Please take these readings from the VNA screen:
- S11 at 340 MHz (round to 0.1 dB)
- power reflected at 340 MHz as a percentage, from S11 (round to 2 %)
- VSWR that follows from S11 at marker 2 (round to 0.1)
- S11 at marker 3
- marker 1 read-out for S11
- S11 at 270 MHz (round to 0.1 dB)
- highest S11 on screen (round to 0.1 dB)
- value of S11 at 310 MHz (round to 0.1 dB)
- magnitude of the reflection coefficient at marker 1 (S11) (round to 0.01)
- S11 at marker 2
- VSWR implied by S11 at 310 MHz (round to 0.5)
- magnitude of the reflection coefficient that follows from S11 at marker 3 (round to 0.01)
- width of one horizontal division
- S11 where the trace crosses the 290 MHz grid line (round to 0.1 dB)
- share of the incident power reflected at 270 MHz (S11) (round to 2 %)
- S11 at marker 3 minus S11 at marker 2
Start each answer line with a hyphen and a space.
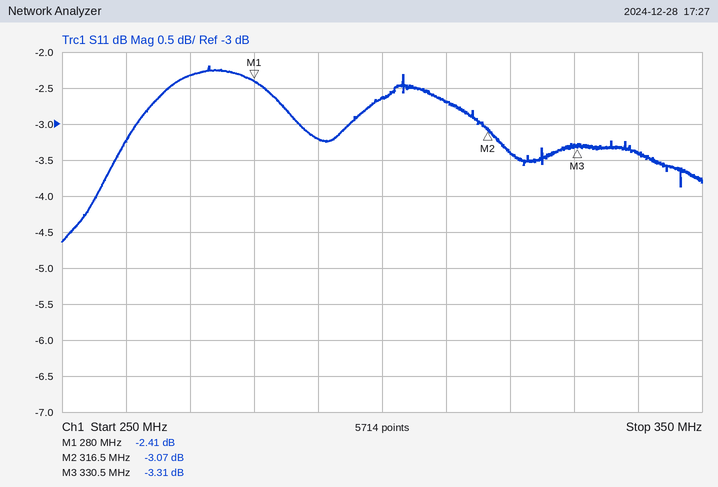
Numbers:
- -3.4 dB
- 46 %
- 5.7
- -3.31 dB
- -2.41 dB
- -2.3 dB
- -2.2 dB
- -2.7 dB
- 0.76
- -3.07 dB
- 6.5
- 0.68
- 10 MHz
- -3.2 dB
- 58 %
- -0.24 dB
